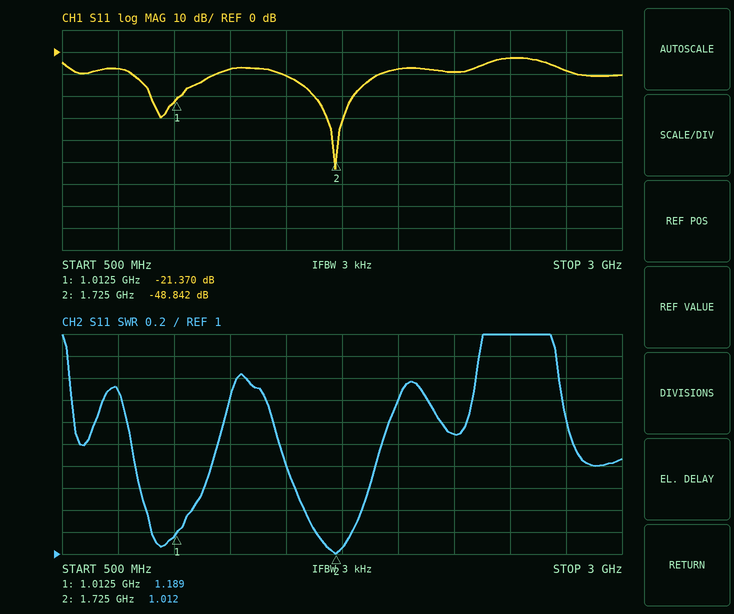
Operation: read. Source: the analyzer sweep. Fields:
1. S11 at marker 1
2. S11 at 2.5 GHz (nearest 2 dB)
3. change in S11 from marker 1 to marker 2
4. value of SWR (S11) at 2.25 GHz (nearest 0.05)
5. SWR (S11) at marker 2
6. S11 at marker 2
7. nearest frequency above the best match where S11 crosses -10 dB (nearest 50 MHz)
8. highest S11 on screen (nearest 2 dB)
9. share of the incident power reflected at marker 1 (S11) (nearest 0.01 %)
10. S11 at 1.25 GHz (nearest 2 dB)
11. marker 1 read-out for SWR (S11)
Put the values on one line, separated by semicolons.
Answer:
-21.370 dB; -2 dB; -27.472 dB; 2.10; 1.012; -48.842 dB; 1.90 GHz; -2 dB; 0.73 %; -8 dB; 1.189
